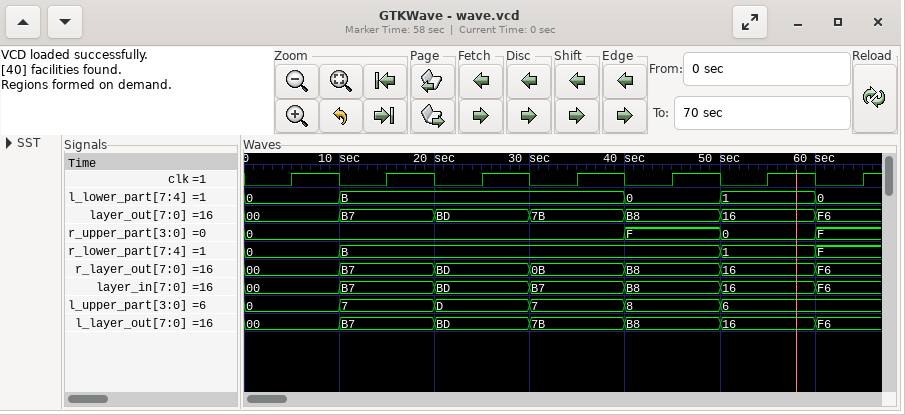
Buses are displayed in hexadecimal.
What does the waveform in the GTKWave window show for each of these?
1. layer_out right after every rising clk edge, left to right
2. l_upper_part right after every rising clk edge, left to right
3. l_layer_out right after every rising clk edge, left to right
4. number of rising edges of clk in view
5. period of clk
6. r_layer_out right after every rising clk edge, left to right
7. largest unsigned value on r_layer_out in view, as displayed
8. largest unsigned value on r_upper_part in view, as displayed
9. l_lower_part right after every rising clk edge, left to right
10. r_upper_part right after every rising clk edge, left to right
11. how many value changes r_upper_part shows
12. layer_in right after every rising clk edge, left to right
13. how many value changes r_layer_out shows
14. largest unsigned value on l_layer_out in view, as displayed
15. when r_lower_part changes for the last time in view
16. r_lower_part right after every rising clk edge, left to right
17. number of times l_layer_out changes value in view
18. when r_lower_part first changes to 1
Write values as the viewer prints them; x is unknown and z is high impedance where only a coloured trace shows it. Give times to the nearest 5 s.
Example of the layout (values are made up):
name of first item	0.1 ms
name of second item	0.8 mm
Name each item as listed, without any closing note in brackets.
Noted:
layer_out right after every rising clk edge, left to right	00, B7, BD, 7B, B8, 16, F6
l_upper_part right after every rising clk edge, left to right	0, 7, D, 7, 8, 6, 6
l_layer_out right after every rising clk edge, left to right	00, B7, BD, 7B, B8, 16, F6
number of rising edges of clk in view	7
period of clk	10 s
r_layer_out right after every rising clk edge, left to right	00, B7, BD, 0B, B8, 16, F6
largest unsigned value on r_layer_out in view, as displayed	F6
largest unsigned value on r_upper_part in view, as displayed	F
l_lower_part right after every rising clk edge, left to right	0, B, B, B, 0, 1, 0
r_upper_part right after every rising clk edge, left to right	0, 0, 0, 0, F, 0, F
how many value changes r_upper_part shows	3
layer_in right after every rising clk edge, left to right	00, B7, BD, B7, B8, 16, F6
how many value changes r_layer_out shows	6
largest unsigned value on l_layer_out in view, as displayed	F6
when r_lower_part changes for the last time in view	60 s
r_lower_part right after every rising clk edge, left to right	0, B, B, B, B, 1, F
number of times l_layer_out changes value in view	6
when r_lower_part first changes to 1	50 s
